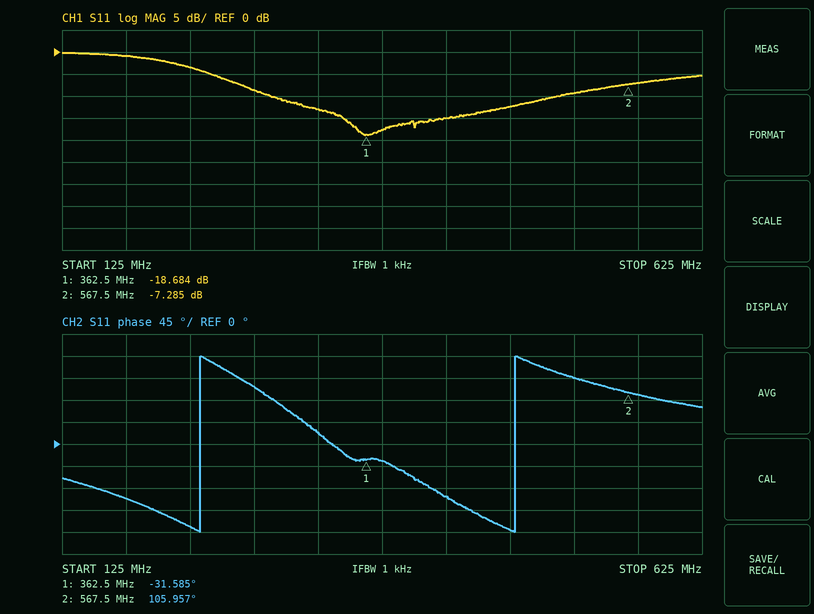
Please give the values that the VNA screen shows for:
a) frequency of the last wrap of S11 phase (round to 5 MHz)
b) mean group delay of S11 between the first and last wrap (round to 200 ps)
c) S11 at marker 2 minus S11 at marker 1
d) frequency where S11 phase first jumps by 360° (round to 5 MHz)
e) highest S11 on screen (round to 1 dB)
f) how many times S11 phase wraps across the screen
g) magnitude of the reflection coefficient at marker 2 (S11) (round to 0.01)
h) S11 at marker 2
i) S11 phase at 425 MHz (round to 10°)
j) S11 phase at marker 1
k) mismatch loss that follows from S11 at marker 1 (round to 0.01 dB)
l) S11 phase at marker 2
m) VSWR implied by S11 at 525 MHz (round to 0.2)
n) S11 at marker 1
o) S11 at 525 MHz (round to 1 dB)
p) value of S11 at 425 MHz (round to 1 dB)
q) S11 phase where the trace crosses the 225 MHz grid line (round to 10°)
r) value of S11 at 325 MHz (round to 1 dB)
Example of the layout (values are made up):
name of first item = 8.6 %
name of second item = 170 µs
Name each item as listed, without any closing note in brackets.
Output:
frequency of the last wrap of S11 phase = 480 MHz
mean group delay of S11 between the first and last wrap = 4.0 ns
S11 at marker 2 minus S11 at marker 1 = 11.399 dB
frequency where S11 phase first jumps by 360° = 235 MHz
highest S11 on screen = 0 dB
how many times S11 phase wraps across the screen = 2
magnitude of the reflection coefficient at marker 2 (S11) = 0.43
S11 at marker 2 = -7.285 dB
S11 phase at 425 MHz = -110°
S11 phase at marker 1 = -31.585°
mismatch loss that follows from S11 at marker 1 = 0.06 dB
S11 phase at marker 2 = 105.957°
VSWR implied by S11 at 525 MHz = 2.0
S11 at marker 1 = -18.684 dB
S11 at 525 MHz = -9 dB
value of S11 at 425 MHz = -15 dB
S11 phase where the trace crosses the 225 MHz grid line = -170°
value of S11 at 325 MHz = -13 dB
